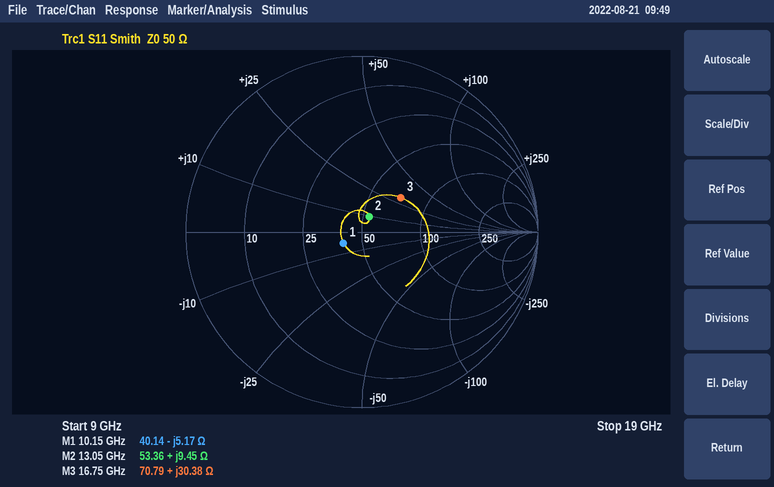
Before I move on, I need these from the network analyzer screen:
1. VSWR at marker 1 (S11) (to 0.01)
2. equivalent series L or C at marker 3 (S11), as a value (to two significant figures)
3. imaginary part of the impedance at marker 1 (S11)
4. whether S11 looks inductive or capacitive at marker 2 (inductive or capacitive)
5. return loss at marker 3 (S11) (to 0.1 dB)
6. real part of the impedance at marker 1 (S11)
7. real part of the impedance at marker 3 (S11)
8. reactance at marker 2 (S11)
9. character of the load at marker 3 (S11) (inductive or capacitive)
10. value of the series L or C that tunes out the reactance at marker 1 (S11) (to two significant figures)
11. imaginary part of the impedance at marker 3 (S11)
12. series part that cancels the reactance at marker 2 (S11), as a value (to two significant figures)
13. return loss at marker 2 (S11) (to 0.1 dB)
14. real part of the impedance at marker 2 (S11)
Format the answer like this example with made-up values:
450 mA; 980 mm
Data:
1.28; 290 pH; -5.17 Ω; inductive; 10.6 dB; 40.14 Ω; 70.79 Ω; +9.45 Ω; inductive; 81 pH; +30.38 Ω; 1.3 pF; 20.3 dB; 53.36 Ω
